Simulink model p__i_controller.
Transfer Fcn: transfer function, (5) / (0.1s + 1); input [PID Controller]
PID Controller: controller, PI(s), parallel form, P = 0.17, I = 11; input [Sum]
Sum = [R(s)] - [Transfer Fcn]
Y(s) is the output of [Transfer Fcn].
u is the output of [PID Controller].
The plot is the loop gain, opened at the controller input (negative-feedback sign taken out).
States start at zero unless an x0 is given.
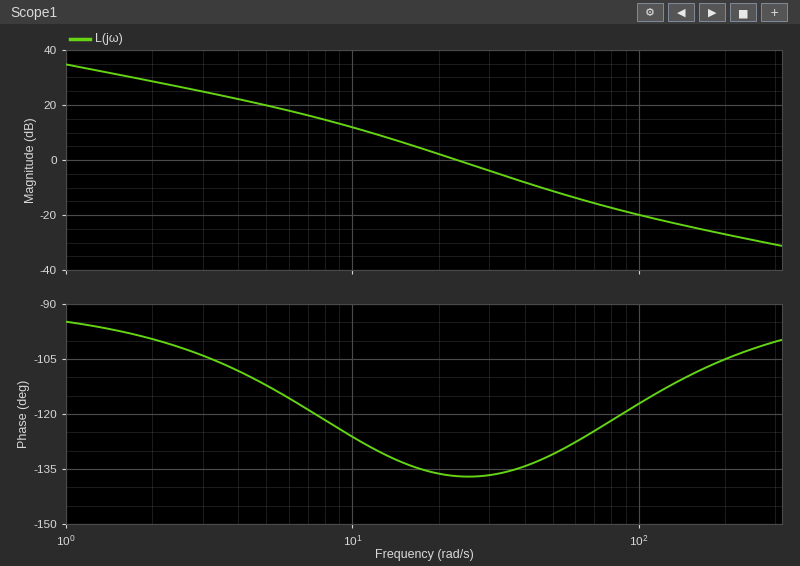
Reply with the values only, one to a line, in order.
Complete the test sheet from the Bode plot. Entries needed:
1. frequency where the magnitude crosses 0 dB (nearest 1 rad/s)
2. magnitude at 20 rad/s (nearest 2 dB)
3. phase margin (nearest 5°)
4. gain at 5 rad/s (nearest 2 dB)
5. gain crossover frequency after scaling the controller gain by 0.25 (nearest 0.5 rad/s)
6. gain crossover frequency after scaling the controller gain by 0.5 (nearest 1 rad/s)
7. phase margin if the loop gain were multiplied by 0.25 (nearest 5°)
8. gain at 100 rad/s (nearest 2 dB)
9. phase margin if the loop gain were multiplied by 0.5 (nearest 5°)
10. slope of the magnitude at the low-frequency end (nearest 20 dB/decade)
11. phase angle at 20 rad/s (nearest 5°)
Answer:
23 rad/s
2 dB
45°
20 dB
10.0 rad/s
15 rad/s
55°
-20 dB
45°
-20 dB/decade
-135°
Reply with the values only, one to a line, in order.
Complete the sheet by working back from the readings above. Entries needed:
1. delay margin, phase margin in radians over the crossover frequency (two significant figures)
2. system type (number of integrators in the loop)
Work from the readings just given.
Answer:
0.034 s
1
